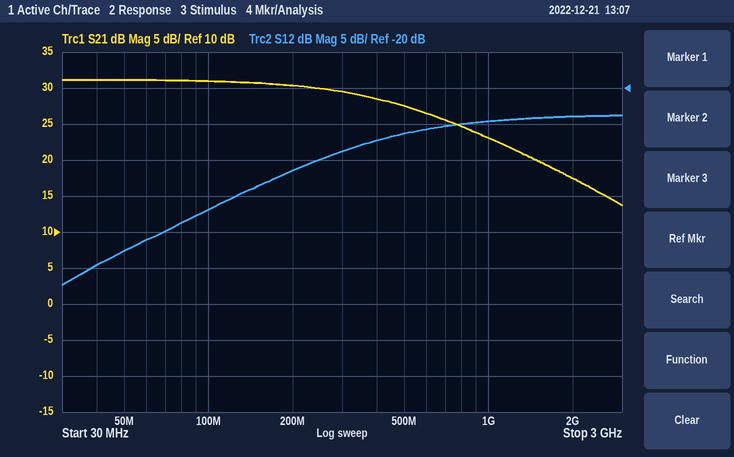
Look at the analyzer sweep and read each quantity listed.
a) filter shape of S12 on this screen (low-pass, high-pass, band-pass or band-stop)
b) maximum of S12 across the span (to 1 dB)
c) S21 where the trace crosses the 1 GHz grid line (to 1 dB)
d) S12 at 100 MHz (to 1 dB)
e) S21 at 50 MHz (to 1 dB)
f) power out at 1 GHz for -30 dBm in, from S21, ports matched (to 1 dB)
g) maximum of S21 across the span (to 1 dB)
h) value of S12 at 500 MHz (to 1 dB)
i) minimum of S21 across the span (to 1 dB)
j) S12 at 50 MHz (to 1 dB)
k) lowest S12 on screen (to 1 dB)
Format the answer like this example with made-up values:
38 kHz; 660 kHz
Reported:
high-pass; -24 dB; 23 dB; -37 dB; 31 dB; -7 dBm; 31 dB; -26 dB; 14 dB; -43 dB; -47 dB
